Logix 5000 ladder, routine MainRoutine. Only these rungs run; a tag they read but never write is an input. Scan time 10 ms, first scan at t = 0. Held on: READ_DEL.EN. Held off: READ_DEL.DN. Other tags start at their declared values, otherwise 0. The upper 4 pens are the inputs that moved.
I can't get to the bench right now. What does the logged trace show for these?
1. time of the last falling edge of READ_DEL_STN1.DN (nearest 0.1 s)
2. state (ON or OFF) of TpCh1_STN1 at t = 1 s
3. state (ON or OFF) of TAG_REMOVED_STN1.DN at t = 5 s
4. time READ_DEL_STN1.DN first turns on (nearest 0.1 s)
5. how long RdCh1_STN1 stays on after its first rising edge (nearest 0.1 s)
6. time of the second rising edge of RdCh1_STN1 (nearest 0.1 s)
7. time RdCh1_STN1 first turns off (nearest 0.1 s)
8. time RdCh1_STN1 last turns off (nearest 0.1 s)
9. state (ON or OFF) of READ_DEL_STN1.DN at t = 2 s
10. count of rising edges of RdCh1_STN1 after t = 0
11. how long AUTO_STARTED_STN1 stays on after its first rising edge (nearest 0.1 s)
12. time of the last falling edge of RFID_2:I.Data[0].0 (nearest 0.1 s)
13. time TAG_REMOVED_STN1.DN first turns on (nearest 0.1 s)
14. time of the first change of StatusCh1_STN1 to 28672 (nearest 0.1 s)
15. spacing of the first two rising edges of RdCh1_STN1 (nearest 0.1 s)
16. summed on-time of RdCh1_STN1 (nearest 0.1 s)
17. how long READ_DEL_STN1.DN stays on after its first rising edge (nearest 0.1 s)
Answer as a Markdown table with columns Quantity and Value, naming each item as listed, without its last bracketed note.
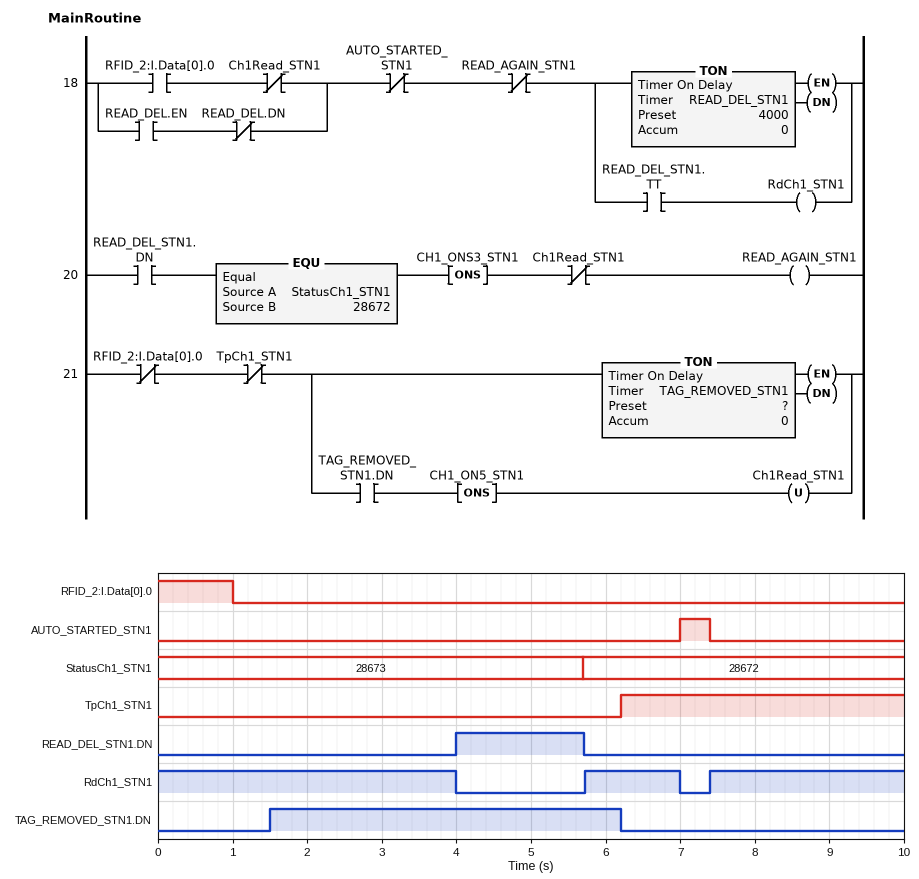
| Quantity | Value |
|---|---|
| time of the last falling edge of READ_DEL_STN1.DN | 5.7 s |
| state (ON or OFF) of TpCh1_STN1 at t = 1 s | OFF |
| state (ON or OFF) of TAG_REMOVED_STN1.DN at t = 5 s | ON |
| time READ_DEL_STN1.DN first turns on | 4.0 s |
| how long RdCh1_STN1 stays on after its first rising edge | 1.3 s |
| time of the second rising edge of RdCh1_STN1 | 7.4 s |
| time RdCh1_STN1 first turns off | 4.0 s |
| time RdCh1_STN1 last turns off | 7.0 s |
| state (ON or OFF) of READ_DEL_STN1.DN at t = 2 s | OFF |
| count of rising edges of RdCh1_STN1 after t = 0 | 2 |
| how long AUTO_STARTED_STN1 stays on after its first rising edge | 0.4 s |
| time of the last falling edge of RFID_2:I.Data[0].0 | 1.0 s |
| time TAG_REMOVED_STN1.DN first turns on | 1.5 s |
| time of the first change of StatusCh1_STN1 to 28672 | 5.7 s |
| spacing of the first two rising edges of RdCh1_STN1 | 1.7 s |
| summed on-time of RdCh1_STN1 | 7.9 s |
| how long READ_DEL_STN1.DN stays on after its first rising edge | 1.7 s |
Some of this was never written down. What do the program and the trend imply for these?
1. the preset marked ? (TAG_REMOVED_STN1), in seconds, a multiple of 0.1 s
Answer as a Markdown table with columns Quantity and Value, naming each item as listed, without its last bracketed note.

| Quantity | Value |
|---|---|
| the preset marked ? (TAG_REMOVED_STN1), in seconds, a multiple of 0.1 s | 0.5 s |
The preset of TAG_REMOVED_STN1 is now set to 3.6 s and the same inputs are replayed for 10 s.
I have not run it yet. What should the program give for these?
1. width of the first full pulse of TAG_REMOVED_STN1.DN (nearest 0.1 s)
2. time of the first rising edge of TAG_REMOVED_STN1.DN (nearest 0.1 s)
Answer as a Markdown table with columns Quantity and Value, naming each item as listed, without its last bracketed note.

| Quantity | Value |
|---|---|
| width of the first full pulse of TAG_REMOVED_STN1.DN | 1.6 s |
| time of the first rising edge of TAG_REMOVED_STN1.DN | 4.6 s |
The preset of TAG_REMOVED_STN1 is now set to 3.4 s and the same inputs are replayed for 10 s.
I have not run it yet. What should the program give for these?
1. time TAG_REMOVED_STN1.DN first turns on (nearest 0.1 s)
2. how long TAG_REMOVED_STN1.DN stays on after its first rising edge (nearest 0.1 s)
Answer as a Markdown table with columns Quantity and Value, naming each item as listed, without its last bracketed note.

| Quantity | Value |
|---|---|
| time TAG_REMOVED_STN1.DN first turns on | 4.4 s |
| how long TAG_REMOVED_STN1.DN stays on after its first rising edge | 1.8 s |
